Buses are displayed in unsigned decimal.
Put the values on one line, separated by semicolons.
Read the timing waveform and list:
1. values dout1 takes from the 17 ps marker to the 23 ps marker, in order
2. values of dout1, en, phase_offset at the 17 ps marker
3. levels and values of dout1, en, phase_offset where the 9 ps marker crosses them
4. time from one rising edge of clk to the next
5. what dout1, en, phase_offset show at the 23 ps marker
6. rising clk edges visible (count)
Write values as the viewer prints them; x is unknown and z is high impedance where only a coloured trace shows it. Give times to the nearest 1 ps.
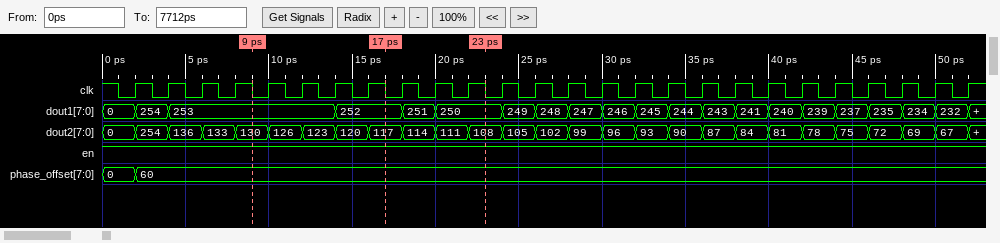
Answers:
252, 251, 250; dout1=252, en=1, phase_offset=60; dout1=253, en=1, phase_offset=60; 2 ps; dout1=250, en=1, phase_offset=60; 26
